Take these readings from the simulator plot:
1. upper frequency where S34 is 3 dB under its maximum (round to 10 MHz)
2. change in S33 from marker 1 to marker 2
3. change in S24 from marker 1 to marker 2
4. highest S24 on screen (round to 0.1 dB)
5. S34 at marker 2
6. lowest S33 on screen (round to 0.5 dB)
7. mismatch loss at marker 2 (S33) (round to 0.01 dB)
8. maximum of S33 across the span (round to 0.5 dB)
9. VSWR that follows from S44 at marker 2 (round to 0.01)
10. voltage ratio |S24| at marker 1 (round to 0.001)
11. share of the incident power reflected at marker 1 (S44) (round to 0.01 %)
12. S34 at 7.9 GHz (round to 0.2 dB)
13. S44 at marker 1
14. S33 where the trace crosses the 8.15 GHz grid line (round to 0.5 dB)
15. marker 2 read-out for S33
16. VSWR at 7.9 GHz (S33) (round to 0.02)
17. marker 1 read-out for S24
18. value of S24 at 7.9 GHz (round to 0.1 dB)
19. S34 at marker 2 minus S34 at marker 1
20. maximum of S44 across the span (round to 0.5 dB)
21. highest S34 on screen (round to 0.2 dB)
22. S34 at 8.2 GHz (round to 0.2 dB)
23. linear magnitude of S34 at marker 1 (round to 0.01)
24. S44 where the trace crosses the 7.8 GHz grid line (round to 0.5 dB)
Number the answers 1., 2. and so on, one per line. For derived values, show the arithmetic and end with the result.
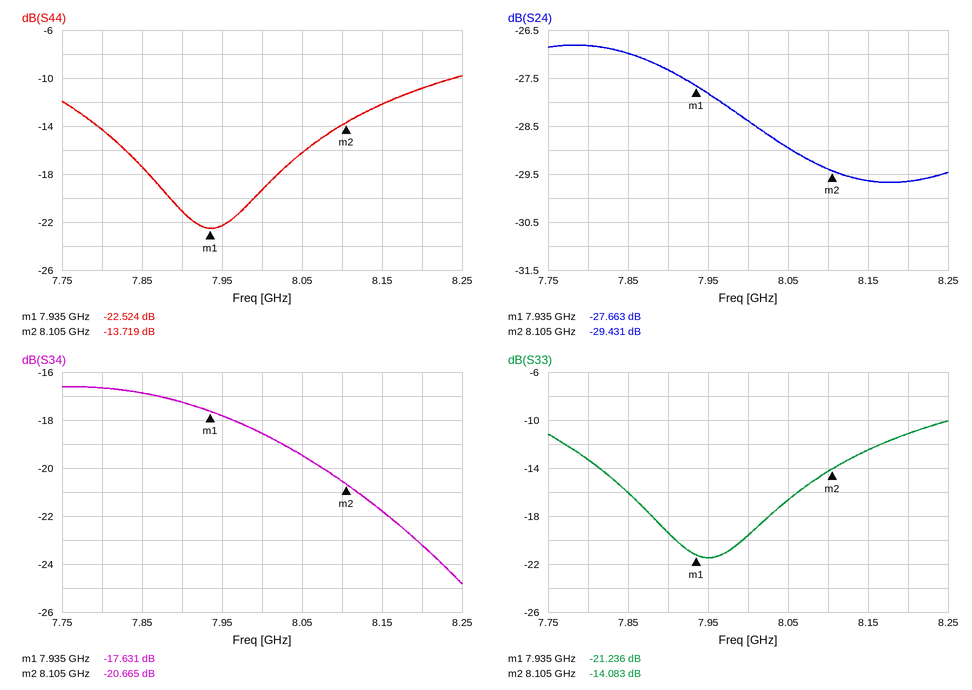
1. 8.06 GHz
2. -14.083 − (-21.236) = 7.153 dB
3. -29.431 − (-27.663) = -1.768 dB
4. -26.8 dB
5. -20.665 dB
6. -21.5 dB
7. −10 log10(1 − 10^(-14.083/10)) ≈ 0.17 dB
8. -10.0 dB
9. (1 + 0.2061)/(1 − 0.2061) ≈ 1.52
10. 10^(-27.663/20) ≈ 0.041
11. 10^(-22.524/10) ≈ 0.56 %
12. -17.2 dB
13. -22.524 dB
14. -12.5 dB
15. -14.083 dB
16. |Γ| = 10^(-19.5/20) = 0.1059; VSWR = (1 + 0.1059)/(1 − 0.1059) ≈ 1.24
17. -27.663 dB
18. -27.3 dB
19. -20.665 − (-17.631) = -3.034 dB
20. -10.0 dB
21. -16.6 dB
22. -23.2 dB
23. 10^(-17.631/20) ≈ 0.13
24. -14.5 dB
